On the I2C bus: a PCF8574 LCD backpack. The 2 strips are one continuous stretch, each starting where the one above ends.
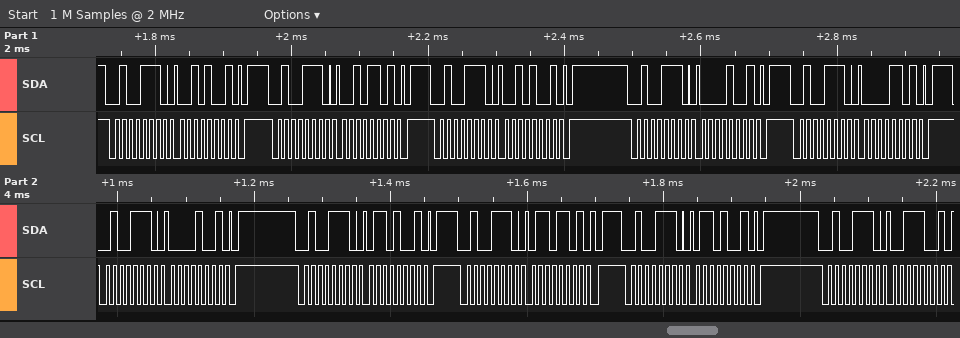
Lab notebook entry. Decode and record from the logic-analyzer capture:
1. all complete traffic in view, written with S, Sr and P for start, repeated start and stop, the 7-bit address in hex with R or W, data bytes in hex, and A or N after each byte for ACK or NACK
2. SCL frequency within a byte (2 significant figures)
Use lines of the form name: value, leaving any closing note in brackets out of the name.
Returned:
all complete traffic in view, written with S, Sr and P for start, repeated start and stop, the 7-bit address in hex with R or W, data bytes in hex, and A or N after each byte for ACK or NACK: S 27W A 29 A P S 27W A 2D A P S 27W A 29 A P S 27W A 09 A P S 27W A 0D A P S 27W A 09 A P S 27W A 69 A P S 27W A 6D A P S 27W A 69 A P S 27W A 39 A
SCL frequency within a byte: 100 kHz
